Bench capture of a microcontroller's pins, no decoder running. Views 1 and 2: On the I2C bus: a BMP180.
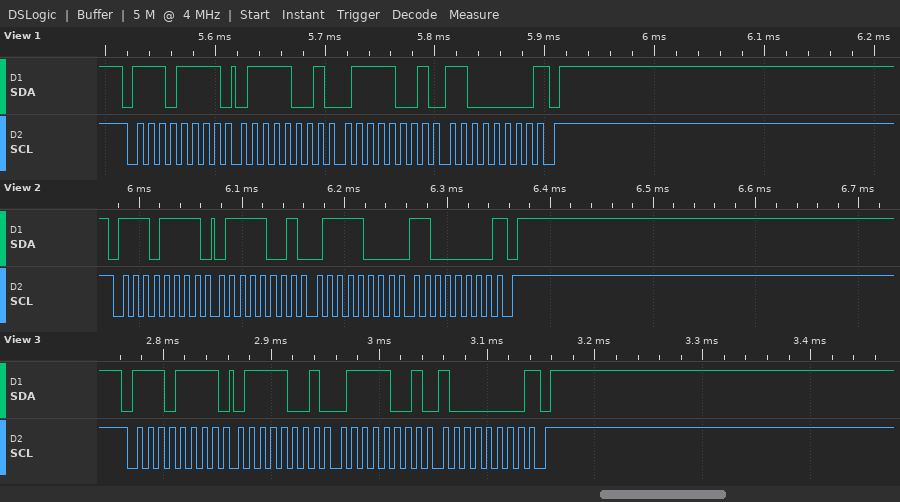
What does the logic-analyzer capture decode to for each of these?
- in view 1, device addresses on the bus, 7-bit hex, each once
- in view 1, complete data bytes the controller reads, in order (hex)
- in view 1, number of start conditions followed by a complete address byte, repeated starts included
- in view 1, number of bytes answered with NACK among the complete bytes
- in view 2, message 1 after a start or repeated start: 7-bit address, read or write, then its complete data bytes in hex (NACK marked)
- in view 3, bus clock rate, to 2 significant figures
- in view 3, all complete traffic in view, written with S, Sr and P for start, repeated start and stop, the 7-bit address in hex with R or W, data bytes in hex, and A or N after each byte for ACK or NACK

0x77
79 79 C0
1
1
0x77 read: 79 78 C0 NACK
100 kHz
S 77R A 79 A 79 A 80 N P
